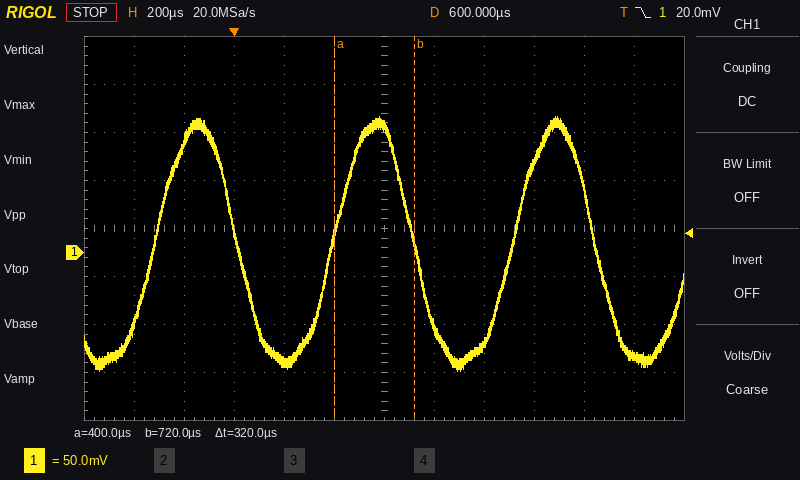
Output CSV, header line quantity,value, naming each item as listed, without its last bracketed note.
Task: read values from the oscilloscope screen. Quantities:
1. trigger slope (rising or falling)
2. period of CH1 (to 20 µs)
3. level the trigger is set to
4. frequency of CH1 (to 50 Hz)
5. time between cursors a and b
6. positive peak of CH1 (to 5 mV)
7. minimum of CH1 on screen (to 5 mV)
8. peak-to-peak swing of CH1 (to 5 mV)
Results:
quantity,value
trigger slope,falling
period of CH1,720 µs
level the trigger is set to,20.0 mV
frequency of CH1,1.40 kHz
time between cursors a and b,320 µs
positive peak of CH1,140 mV
minimum of CH1 on screen,-125 mV
peak-to-peak swing of CH1,265 mV
